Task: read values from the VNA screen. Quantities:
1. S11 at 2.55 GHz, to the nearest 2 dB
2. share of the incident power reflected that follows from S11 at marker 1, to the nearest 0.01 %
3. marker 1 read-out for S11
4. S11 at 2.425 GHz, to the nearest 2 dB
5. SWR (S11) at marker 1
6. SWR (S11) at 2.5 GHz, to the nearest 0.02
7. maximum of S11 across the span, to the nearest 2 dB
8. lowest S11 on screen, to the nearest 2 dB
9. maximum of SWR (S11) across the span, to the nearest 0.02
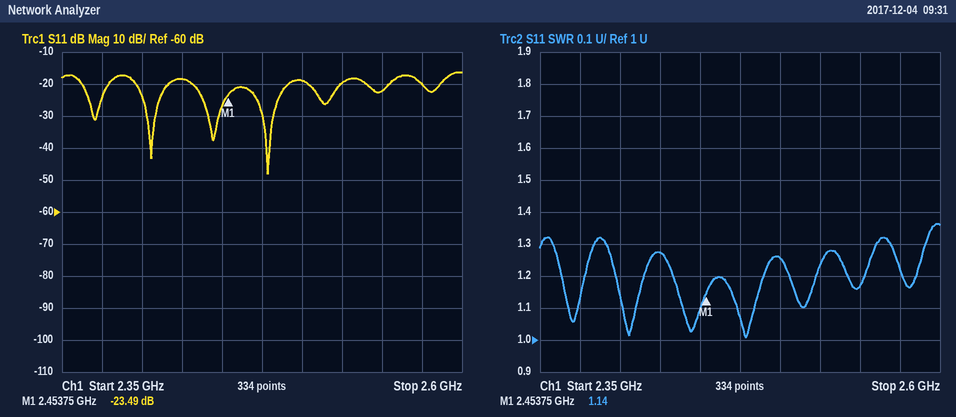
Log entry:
-22 dB
0.45 %
-23.49 dB
-18 dB
1.14
1.26
-16 dB
-48 dB
1.36
